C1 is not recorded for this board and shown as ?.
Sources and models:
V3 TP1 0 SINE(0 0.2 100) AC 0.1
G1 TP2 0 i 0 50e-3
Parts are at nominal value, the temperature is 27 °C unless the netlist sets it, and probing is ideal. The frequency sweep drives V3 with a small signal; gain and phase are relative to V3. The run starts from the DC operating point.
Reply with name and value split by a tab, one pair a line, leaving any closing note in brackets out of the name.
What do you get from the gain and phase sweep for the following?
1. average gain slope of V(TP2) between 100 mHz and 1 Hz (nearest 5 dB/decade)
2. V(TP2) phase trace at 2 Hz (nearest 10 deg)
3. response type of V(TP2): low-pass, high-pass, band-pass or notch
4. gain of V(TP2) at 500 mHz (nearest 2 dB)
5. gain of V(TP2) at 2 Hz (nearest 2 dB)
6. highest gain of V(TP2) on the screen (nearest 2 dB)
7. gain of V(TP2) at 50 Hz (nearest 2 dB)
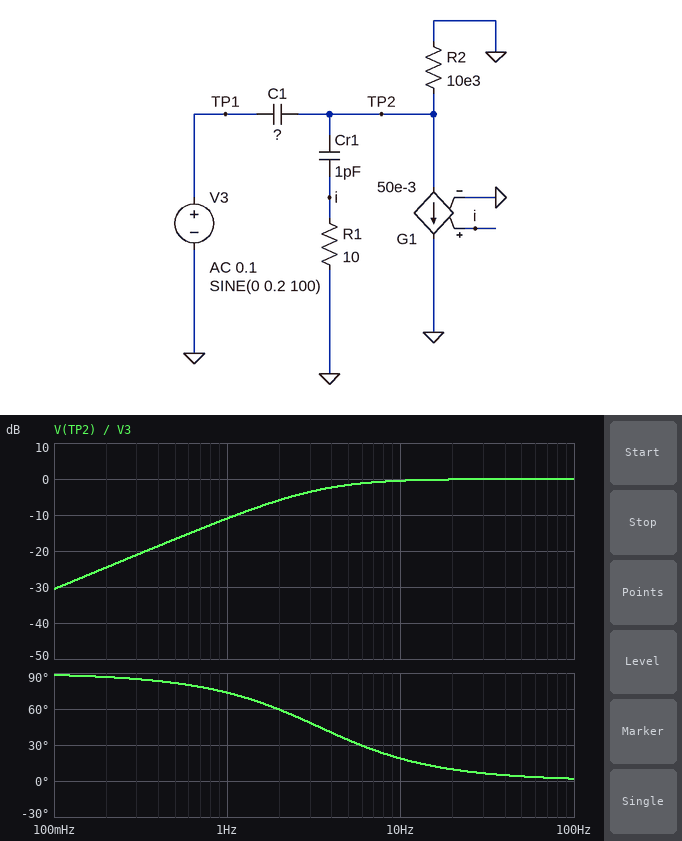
average gain slope of V(TP2) between 100 mHz and 1 Hz	20 dB/decade
V(TP2) phase trace at 2 Hz	60 deg
response type of V(TP2): low-pass, high-pass, band-pass or notch	high-pass
gain of V(TP2) at 500 mHz	-16 dB
gain of V(TP2) at 2 Hz	-6 dB
highest gain of V(TP2) on the screen	0 dB
gain of V(TP2) at 50 Hz	0 dB
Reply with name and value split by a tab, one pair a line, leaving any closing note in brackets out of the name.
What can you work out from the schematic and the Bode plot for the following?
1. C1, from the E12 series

C1, from the E12 series	4.7 µF
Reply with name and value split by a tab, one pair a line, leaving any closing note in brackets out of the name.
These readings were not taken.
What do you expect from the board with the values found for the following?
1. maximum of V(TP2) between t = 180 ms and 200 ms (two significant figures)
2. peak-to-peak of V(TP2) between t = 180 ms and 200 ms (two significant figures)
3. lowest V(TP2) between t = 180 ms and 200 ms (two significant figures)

maximum of V(TP2) between t = 180 ms and 200 ms	200 mV
peak-to-peak of V(TP2) between t = 180 ms and 200 ms	400 mV
lowest V(TP2) between t = 180 ms and 200 ms	-200 mV
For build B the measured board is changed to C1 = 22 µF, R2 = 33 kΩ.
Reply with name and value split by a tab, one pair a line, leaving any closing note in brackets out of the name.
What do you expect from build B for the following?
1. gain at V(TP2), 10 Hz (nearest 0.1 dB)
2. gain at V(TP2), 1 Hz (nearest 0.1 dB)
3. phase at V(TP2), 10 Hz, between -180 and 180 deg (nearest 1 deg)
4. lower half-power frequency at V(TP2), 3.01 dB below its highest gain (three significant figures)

gain at V(TP2), 10 Hz	0 dB
gain at V(TP2), 1 Hz	-0.2 dB
phase at V(TP2), 10 Hz, between -180 and 180 deg	1 deg
lower half-power frequency at V(TP2), 3.01 dB below its highest gain	219 mHz
